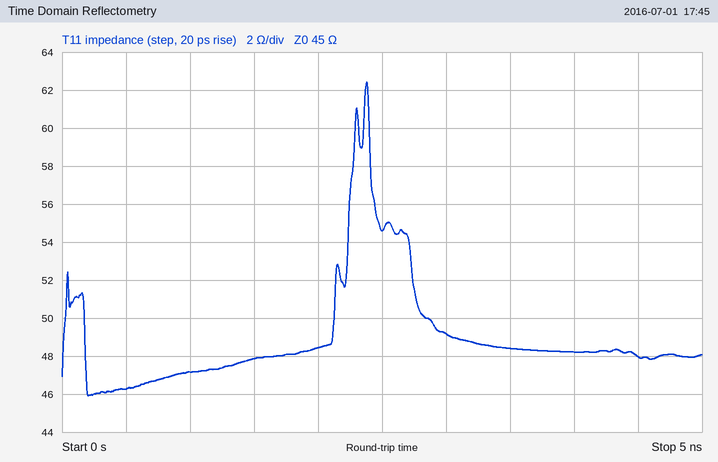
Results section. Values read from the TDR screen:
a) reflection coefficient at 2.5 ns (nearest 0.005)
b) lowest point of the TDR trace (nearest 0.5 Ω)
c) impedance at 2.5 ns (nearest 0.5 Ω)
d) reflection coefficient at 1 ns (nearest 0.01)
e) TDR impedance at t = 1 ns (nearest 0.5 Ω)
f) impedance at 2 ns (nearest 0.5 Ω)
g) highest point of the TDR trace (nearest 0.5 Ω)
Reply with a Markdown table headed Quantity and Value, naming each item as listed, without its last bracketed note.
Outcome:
| Quantity | Value |
|---|---|
| reflection coefficient at 2.5 ns | +0.095 |
| lowest point of the TDR trace | 46.0 Ω |
| impedance at 2.5 ns | 54.5 Ω |
| reflection coefficient at 1 ns | +0.02 |
| TDR impedance at t = 1 ns | 47.0 Ω |
| impedance at 2 ns | 48.5 Ω |
| highest point of the TDR trace | 62.5 Ω |
